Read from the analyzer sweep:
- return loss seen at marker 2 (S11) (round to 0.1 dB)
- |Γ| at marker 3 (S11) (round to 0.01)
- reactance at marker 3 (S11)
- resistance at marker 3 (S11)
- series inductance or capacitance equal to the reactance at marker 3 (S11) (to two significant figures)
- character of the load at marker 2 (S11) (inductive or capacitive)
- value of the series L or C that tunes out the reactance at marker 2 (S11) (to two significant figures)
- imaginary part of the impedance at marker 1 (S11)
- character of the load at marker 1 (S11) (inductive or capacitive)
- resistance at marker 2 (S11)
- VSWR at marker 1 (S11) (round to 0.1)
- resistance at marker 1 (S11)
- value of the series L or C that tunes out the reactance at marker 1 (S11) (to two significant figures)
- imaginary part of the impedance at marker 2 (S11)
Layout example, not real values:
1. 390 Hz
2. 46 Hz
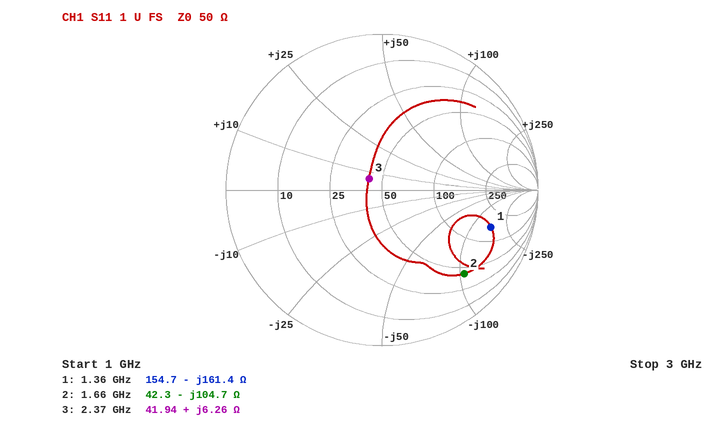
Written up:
1. 2.5 dB
2. 0.11
3. +6.26 Ω
4. 41.94 Ω
5. 420 pH
6. capacitive
7. 10 nH
8. -161.4 Ω
9. capacitive
10. 42.3 Ω
11. 6.6
12. 154.7 Ω
13. 19 nH
14. -104.7 Ω
